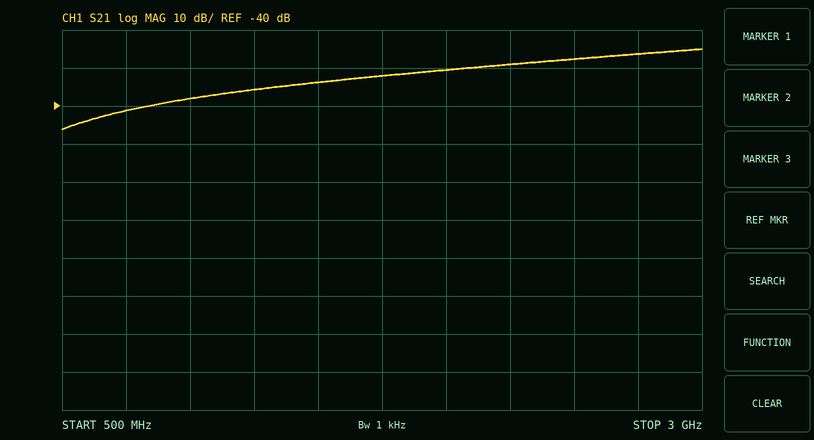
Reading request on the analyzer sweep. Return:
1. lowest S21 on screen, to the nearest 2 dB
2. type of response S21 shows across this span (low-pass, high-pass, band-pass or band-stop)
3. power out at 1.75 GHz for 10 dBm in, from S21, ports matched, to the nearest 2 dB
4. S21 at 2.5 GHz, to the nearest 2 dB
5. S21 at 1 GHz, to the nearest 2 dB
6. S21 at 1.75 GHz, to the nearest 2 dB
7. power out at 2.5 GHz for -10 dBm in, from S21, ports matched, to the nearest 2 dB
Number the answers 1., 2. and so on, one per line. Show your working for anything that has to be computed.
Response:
1. -46 dB
2. high-pass
3. 10 dBm + (-32 dB) = -22 dBm
4. -28 dB
5. -38 dB
6. -32 dB
7. -10 dBm + (-28 dB) = -38 dBm
